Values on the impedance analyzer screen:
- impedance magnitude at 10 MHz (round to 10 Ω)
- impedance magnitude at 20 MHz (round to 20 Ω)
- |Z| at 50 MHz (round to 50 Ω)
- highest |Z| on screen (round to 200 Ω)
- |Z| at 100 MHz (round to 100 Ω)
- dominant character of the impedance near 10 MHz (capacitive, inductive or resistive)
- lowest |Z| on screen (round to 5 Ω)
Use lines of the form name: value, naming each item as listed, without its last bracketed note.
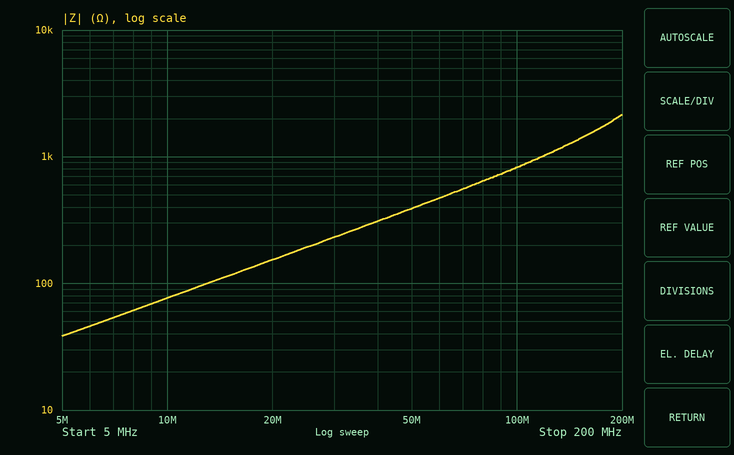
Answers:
impedance magnitude at 10 MHz: 80 Ω
impedance magnitude at 20 MHz: 160 Ω
|Z| at 50 MHz: 400 Ω
highest |Z| on screen: 2.2 kΩ
|Z| at 100 MHz: 800 Ω
dominant character of the impedance near 10 MHz: inductive
lowest |Z| on screen: 40 Ω
